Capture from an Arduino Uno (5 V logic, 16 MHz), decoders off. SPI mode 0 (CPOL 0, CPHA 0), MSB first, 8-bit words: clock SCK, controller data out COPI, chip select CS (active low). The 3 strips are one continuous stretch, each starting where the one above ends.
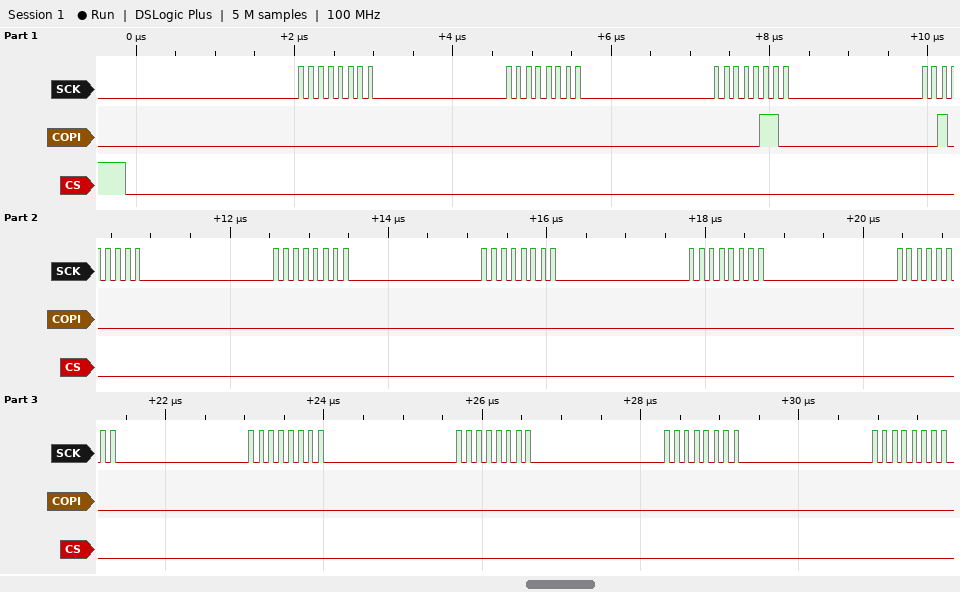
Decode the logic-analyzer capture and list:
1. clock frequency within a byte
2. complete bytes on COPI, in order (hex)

8 MHz
00 00 06 20 00 00 00 00 00 00 00 00
